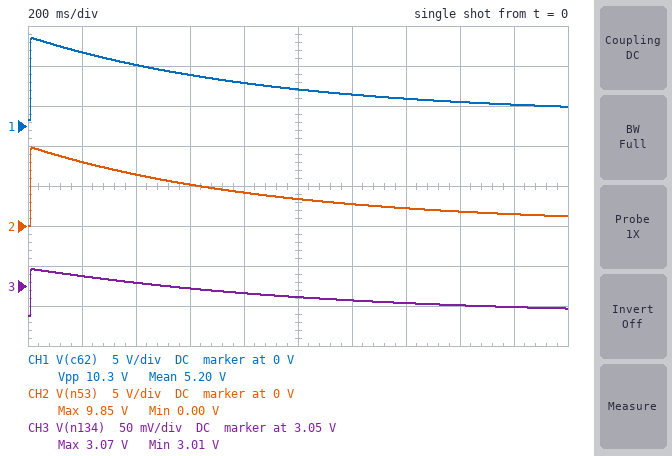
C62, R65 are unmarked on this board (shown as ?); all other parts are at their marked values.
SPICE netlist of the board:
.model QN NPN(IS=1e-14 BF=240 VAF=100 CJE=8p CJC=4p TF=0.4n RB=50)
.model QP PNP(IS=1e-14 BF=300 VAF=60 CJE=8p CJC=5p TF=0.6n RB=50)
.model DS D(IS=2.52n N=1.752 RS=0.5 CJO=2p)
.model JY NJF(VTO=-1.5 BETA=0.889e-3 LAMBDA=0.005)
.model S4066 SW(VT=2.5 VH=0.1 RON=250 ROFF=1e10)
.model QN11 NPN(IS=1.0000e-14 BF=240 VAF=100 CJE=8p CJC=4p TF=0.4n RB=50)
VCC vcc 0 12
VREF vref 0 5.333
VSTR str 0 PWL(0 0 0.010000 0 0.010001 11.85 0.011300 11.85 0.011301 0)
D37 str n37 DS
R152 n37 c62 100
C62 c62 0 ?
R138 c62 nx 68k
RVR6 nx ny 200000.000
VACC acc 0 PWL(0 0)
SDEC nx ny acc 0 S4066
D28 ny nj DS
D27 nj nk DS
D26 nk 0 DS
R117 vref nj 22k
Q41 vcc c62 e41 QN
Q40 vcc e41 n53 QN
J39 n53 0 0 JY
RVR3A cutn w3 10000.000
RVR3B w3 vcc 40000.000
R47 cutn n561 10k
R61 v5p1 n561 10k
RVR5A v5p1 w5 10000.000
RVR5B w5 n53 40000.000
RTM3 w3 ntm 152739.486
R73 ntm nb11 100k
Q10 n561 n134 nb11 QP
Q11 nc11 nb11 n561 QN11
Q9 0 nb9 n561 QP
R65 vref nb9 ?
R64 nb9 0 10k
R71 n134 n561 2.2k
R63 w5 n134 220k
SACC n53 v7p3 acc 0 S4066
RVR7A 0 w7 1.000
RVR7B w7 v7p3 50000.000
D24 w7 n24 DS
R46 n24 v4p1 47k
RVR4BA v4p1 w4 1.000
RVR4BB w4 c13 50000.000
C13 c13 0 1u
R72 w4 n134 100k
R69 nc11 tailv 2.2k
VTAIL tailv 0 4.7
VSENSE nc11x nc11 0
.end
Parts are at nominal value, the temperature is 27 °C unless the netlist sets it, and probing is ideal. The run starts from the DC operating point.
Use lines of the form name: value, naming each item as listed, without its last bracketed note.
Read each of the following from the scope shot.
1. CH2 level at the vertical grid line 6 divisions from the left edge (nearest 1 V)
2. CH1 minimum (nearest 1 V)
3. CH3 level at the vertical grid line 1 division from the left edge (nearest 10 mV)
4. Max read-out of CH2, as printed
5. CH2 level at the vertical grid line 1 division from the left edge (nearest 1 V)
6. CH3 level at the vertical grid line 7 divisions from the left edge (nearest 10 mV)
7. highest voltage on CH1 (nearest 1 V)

CH2 level at the vertical grid line 6 divisions from the left edge: 3 V
CH1 minimum: 1 V
CH3 level at the vertical grid line 1 division from the left edge: 3.06 V
Max read-out of CH2, as printed: 9.85 V
CH2 level at the vertical grid line 1 division from the left edge: 8 V
CH3 level at the vertical grid line 7 divisions from the left edge: 3.03 V
highest voltage on CH1: 11 V
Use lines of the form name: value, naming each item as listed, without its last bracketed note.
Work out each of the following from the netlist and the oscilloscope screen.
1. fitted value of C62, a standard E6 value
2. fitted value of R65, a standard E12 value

fitted value of C62, a standard E6 value: 3.3 µF
fitted value of R65, a standard E12 value: 12 kΩ
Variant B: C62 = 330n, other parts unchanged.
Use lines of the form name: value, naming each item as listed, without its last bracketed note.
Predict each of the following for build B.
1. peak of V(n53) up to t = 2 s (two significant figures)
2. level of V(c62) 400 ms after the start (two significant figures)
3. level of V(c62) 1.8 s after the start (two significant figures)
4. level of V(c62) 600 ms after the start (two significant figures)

peak of V(n53) up to t = 2 s: 10 V
level of V(c62) 400 ms after the start: 1.4 V
level of V(c62) 1.8 s after the start: 1.1 V
level of V(c62) 600 ms after the start: 1.2 V
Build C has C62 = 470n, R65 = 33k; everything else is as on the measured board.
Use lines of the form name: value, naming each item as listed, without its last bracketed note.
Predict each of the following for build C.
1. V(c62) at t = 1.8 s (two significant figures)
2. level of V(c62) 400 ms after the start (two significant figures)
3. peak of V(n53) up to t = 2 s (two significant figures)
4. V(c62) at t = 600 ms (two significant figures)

V(c62) at t = 1.8 s: 1.1 V
level of V(c62) 400 ms after the start: 1.8 V
peak of V(n53) up to t = 2 s: 10 V
V(c62) at t = 600 ms: 1.4 V
